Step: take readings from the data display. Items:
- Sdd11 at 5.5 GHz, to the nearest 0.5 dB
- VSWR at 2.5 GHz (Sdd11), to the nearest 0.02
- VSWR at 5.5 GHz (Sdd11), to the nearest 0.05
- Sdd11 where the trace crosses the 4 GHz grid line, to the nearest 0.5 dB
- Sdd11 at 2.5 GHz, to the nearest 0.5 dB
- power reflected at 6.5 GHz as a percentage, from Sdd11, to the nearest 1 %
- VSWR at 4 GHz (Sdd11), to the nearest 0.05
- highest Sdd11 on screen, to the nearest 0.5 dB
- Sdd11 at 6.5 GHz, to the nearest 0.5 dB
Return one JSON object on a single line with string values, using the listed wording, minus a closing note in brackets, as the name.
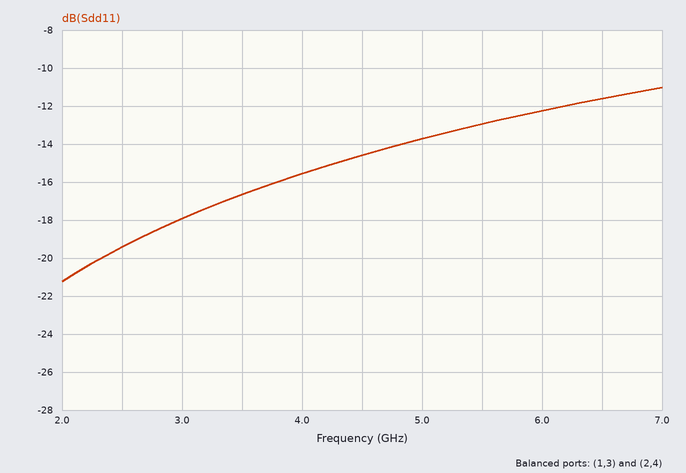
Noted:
{"Sdd11 at 5.5 GHz, to the nearest 0.5 dB": "-13.0 dB", "VSWR at 2.5 GHz (Sdd11), to the nearest 0.02": "1.24", "VSWR at 5.5 GHz (Sdd11), to the nearest 0.05": "1.60", "Sdd11 where the trace crosses the 4 GHz grid line, to the nearest 0.5 dB": "-15.5 dB", "Sdd11 at 2.5 GHz, to the nearest 0.5 dB": "-19.5 dB", "power reflected at 6.5 GHz as a percentage, from Sdd11, to the nearest 1 %": "7 %", "VSWR at 4 GHz (Sdd11), to the nearest 0.05": "1.40", "highest Sdd11 on screen, to the nearest 0.5 dB": "-11.0 dB", "Sdd11 at 6.5 GHz, to the nearest 0.5 dB": "-11.5 dB"}
